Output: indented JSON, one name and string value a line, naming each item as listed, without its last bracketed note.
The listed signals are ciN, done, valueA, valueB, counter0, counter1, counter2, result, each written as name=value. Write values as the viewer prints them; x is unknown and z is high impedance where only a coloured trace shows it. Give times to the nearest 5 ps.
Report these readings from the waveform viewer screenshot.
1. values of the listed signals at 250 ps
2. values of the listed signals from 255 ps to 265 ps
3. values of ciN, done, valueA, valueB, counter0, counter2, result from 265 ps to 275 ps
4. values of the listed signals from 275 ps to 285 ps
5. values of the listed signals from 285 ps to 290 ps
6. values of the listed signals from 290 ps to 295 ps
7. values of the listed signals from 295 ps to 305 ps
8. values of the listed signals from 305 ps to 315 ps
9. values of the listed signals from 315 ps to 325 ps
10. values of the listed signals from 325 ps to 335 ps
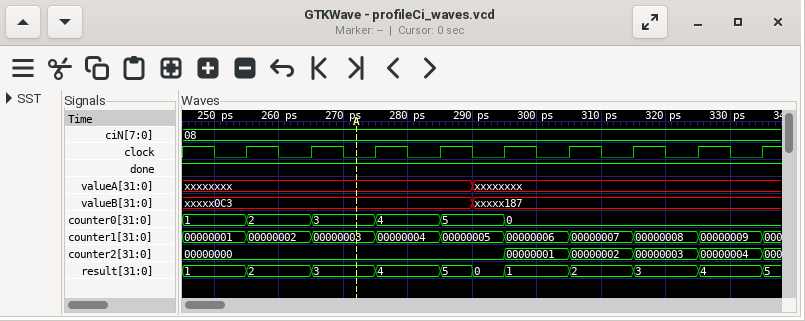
{
  "values of the listed signals at 250 ps": "ciN=08, done=1, valueA=xxxxxxxx, valueB=xxxxx0C3, counter0=1, counter1=00000001, counter2=00000000, result=1",
  "values of the listed signals from 255 ps to 265 ps": "ciN=08, done=1, valueA=xxxxxxxx, valueB=xxxxx0C3, counter0=2, counter1=00000002, counter2=00000000, result=2",
  "values of ciN, done, valueA, valueB, counter0, counter2, result from 265 ps to 275 ps": "ciN=08, done=1, valueA=xxxxxxxx, valueB=xxxxx0C3, counter0=3, counter2=00000000, result=3",
  "values of the listed signals from 275 ps to 285 ps": "ciN=08, done=1, valueA=xxxxxxxx, valueB=xxxxx0C3, counter0=4, counter1=00000004, counter2=00000000, result=4",
  "values of the listed signals from 285 ps to 290 ps": "ciN=08, done=1, valueA=xxxxxxxx, valueB=xxxxx0C3, counter0=5, counter1=00000005, counter2=00000000, result=5",
  "values of the listed signals from 290 ps to 295 ps": "ciN=08, done=1, valueA=xxxxxxxx, valueB=xxxxx187, counter0=5, counter1=00000005, counter2=00000000, result=0",
  "values of the listed signals from 295 ps to 305 ps": "ciN=08, done=1, valueA=xxxxxxxx, valueB=xxxxx187, counter0=0, counter1=00000006, counter2=00000001, result=1",
  "values of the listed signals from 305 ps to 315 ps": "ciN=08, done=1, valueA=xxxxxxxx, valueB=xxxxx187, counter0=0, counter1=00000007, counter2=00000002, result=2",
  "values of the listed signals from 315 ps to 325 ps": "ciN=08, done=1, valueA=xxxxxxxx, valueB=xxxxx187, counter0=0, counter1=00000008, counter2=00000003, result=3",
  "values of the listed signals from 325 ps to 335 ps": "ciN=08, done=1, valueA=xxxxxxxx, valueB=xxxxx187, counter0=0, counter1=00000009, counter2=00000004, result=4"
}
